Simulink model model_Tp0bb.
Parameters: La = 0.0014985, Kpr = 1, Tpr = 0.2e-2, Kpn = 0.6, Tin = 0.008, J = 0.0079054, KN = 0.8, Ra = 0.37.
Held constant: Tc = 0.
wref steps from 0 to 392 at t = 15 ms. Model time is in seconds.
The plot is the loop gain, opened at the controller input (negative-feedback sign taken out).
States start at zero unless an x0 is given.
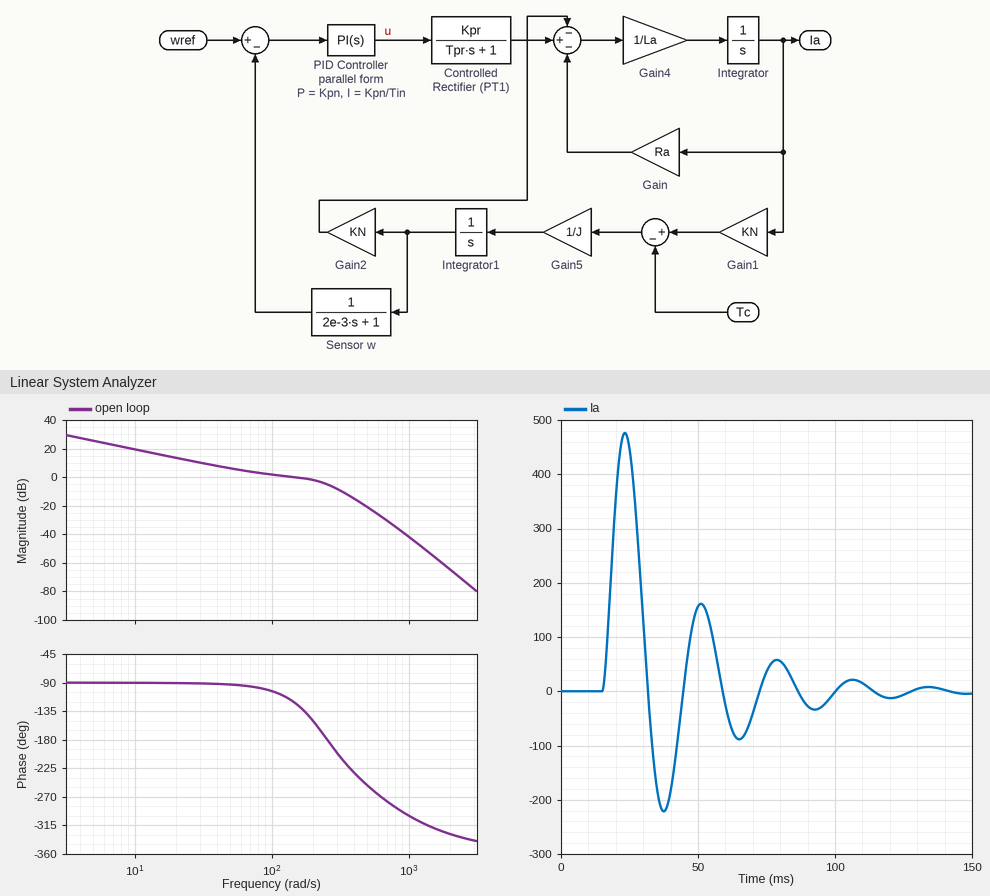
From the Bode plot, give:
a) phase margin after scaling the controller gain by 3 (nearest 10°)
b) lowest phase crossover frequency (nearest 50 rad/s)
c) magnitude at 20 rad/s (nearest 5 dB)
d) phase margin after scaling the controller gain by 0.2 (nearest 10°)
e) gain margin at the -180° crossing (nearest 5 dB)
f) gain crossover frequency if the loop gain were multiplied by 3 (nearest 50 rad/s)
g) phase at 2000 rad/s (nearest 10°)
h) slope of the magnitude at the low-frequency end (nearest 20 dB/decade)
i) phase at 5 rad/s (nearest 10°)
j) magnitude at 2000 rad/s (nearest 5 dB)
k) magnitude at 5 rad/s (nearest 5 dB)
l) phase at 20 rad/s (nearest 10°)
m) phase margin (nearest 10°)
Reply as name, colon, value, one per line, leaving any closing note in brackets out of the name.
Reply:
phase margin after scaling the controller gain by 3: -30°
lowest phase crossover frequency: 250 rad/s
magnitude at 20 rad/s: 15 dB
phase margin after scaling the controller gain by 0.2: 90°
gain margin at the -180° crossing: 5 dB
gain crossover frequency if the loop gain were multiplied by 3: 300 rad/s
phase at 2000 rad/s: -330°
slope of the magnitude at the low-frequency end: -20 dB/decade
phase at 5 rad/s: -90°
magnitude at 2000 rad/s: -65 dB
magnitude at 5 rad/s: 25 dB
phase at 20 rad/s: -90°
phase margin: 60°
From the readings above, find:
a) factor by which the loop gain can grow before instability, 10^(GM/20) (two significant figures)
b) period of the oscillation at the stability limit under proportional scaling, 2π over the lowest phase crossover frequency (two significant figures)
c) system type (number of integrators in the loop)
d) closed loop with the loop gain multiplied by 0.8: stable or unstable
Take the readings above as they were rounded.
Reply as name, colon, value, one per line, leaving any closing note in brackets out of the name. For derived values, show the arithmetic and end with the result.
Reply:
factor by which the loop gain can grow before instability, 10^(GM/20): 10^(5 / 20) = 1.8
period of the oscillation at the stability limit under proportional scaling, 2π over the lowest phase crossover frequency: 2π / 250 = 0.025 s
system type: 1
closed loop with the loop gain multiplied by 0.8: stable or unstable: stable
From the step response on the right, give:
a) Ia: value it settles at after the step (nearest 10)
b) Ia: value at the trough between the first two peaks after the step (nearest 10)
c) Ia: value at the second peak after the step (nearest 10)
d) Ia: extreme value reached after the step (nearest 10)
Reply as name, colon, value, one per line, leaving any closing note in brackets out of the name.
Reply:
Ia: value it settles at after the step: 0
Ia: value at the trough between the first two peaks after the step: -220
Ia: value at the second peak after the step: 160
Ia: extreme value reached after the step: 480
